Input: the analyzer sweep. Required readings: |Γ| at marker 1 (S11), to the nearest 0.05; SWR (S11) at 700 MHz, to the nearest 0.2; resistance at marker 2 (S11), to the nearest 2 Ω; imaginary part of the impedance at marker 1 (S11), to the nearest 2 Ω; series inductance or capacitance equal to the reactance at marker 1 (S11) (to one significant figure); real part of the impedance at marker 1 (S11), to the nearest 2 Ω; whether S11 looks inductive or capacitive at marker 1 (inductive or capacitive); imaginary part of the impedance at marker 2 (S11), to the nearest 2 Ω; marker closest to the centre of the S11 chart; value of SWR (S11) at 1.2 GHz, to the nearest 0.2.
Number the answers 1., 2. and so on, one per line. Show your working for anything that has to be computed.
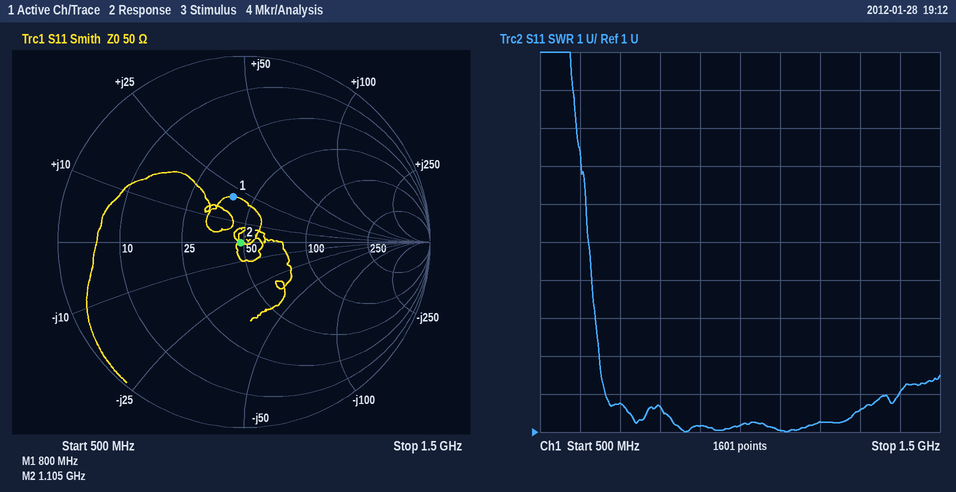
1. 0.25
2. 1.8
3. 48 Ω
4. +20 Ω
5. L = 20 Ω/(2π × 800 MHz) ≈ 4 nH
6. 40 Ω
7. inductive
8. 0 Ω
9. marker 2
10. 1.2
